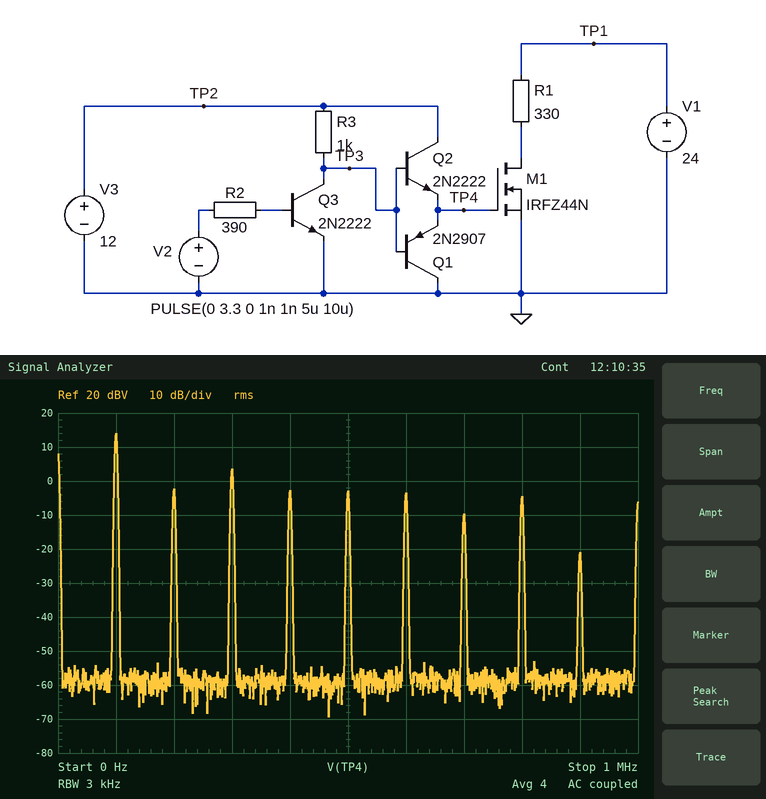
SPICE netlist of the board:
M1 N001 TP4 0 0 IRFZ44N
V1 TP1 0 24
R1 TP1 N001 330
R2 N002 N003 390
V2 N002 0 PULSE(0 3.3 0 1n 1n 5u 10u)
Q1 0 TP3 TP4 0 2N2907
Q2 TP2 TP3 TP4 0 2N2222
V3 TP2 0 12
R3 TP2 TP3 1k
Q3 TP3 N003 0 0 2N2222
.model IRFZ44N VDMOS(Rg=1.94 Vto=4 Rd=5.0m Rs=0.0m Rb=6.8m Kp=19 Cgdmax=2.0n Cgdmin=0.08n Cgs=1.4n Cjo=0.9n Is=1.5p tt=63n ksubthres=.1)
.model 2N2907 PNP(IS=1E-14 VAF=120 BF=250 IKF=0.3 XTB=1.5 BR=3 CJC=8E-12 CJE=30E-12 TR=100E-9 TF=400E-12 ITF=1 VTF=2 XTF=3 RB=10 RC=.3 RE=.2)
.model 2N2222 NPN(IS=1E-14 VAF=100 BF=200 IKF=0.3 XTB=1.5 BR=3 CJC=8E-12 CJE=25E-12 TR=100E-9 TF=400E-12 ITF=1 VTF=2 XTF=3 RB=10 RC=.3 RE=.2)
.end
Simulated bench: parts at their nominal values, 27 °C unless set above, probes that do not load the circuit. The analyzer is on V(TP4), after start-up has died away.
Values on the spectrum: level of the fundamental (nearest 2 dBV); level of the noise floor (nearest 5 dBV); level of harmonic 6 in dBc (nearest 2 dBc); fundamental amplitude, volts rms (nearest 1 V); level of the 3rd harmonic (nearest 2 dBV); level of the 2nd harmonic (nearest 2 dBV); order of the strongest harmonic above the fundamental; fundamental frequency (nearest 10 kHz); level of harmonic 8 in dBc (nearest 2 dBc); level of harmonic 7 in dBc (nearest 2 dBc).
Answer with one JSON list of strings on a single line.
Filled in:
["14 dBV", "-60 dBV", "-18 dBc", "5 V", "4 dBV", "-2 dBV", "3", "100 kHz", "-18 dBc", "-24 dBc"]
